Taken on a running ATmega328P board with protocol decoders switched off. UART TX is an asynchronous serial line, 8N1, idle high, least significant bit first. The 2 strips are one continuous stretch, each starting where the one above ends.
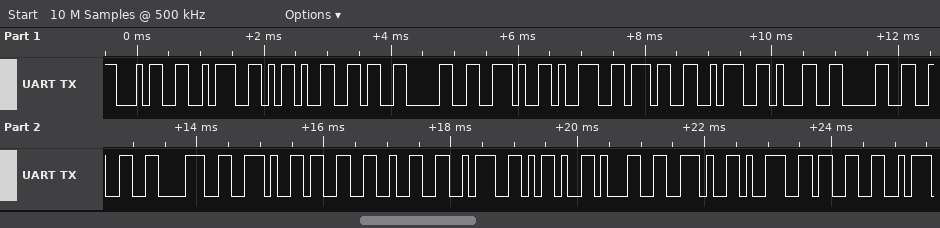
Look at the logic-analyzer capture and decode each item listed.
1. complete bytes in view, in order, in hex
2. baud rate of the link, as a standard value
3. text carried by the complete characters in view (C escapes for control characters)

34 3A 2D 36 30 2E 39 37 3A 31 30 32 38 2E 33 32 3A 2D 31 2E 39 33
9600 baud
"4:-60.97:1028.32:-1.93"
